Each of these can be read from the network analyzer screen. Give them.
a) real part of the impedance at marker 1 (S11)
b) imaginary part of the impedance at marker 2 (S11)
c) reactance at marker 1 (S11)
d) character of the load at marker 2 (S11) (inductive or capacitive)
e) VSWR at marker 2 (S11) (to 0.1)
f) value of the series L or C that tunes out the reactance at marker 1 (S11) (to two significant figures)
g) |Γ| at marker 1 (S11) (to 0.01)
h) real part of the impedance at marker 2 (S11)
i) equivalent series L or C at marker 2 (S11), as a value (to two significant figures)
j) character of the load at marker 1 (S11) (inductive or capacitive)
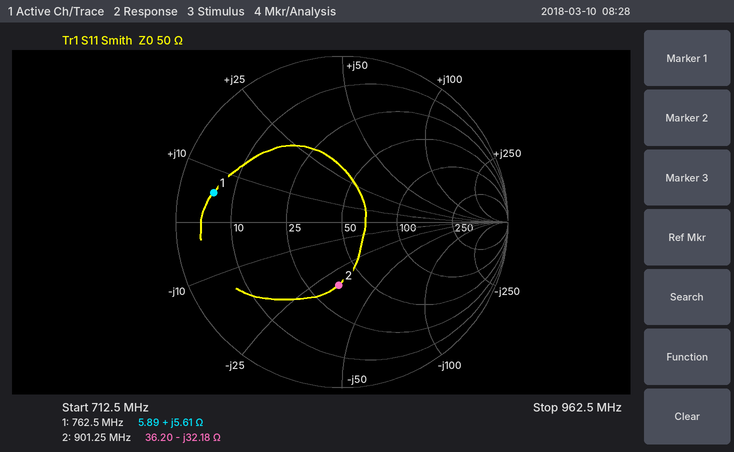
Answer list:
5.89 Ω
-32.18 Ω
+5.61 Ω
capacitive
2.2
37 pF
0.79
36.20 Ω
5.5 pF
inductive
